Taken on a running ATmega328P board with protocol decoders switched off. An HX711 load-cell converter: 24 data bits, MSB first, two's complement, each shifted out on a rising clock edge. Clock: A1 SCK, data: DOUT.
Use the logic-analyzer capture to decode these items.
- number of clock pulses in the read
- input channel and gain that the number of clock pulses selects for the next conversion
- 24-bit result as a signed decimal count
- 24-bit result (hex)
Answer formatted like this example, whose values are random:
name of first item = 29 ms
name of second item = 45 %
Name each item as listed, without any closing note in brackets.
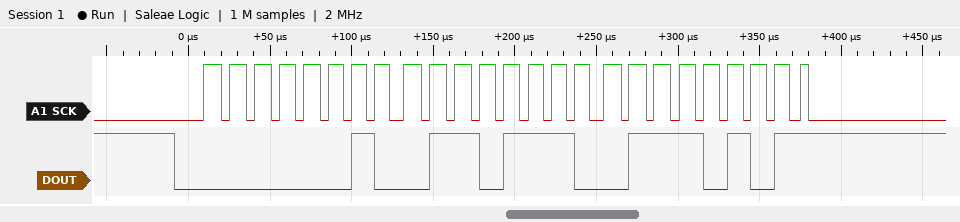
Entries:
number of clock pulses in the read = 25
input channel and gain that the number of clock pulses selects for the next conversion = channel A, gain 128
24-bit result as a signed decimal count = 159349
24-bit result = 0x026E75
